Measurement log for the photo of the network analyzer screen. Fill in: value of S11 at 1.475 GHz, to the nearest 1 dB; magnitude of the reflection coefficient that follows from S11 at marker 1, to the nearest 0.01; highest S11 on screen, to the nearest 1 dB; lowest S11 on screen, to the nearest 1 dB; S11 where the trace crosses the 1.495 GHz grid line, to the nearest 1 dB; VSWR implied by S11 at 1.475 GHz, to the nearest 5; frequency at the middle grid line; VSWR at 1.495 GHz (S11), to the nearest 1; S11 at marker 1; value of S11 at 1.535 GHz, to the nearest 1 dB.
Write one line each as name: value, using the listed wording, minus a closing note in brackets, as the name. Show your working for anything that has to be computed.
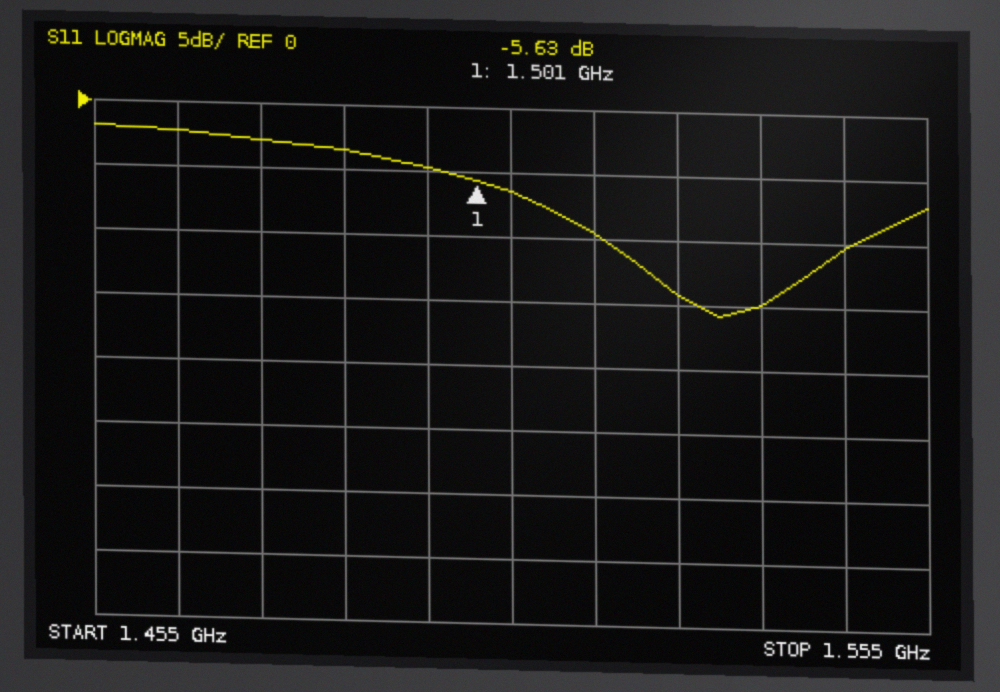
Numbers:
value of S11 at 1.475 GHz, to the nearest 1 dB: -3 dB
magnitude of the reflection coefficient that follows from S11 at marker 1, to the nearest 0.01: 10^(-5.63/20) ≈ 0.52
highest S11 on screen, to the nearest 1 dB: -2 dB
lowest S11 on screen, to the nearest 1 dB: -16 dB
S11 where the trace crosses the 1.495 GHz grid line, to the nearest 1 dB: -5 dB
VSWR implied by S11 at 1.475 GHz, to the nearest 5: |Γ| = 10^(-3/20) = 0.7079; VSWR = (1 + 0.7079)/(1 − 0.7079) ≈ 5.85, so 5 to the nearest 5
frequency at the middle grid line: 1.505 GHz
VSWR at 1.495 GHz (S11), to the nearest 1: |Γ| = 10^(-5/20) = 0.5623; VSWR = (1 + 0.5623)/(1 − 0.5623) ≈ 4
S11 at marker 1: -5.63 dB
value of S11 at 1.535 GHz, to the nearest 1 dB: -15 dB
